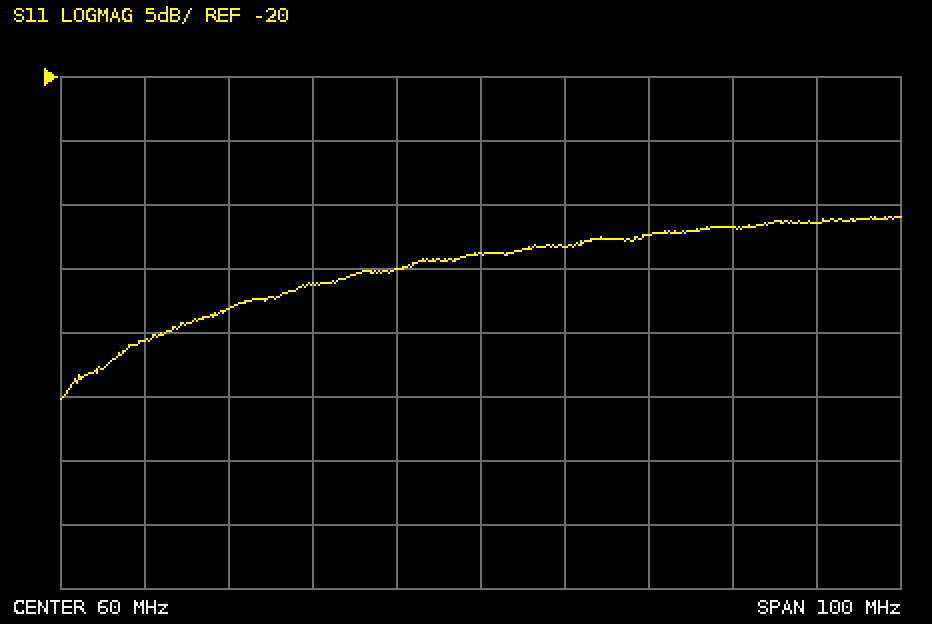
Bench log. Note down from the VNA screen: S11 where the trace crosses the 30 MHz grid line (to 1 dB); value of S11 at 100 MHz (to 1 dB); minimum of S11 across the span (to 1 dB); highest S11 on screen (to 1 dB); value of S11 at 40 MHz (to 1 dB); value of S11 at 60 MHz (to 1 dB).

-38 dB
-31 dB
-45 dB
-31 dB
-36 dB
-34 dB
